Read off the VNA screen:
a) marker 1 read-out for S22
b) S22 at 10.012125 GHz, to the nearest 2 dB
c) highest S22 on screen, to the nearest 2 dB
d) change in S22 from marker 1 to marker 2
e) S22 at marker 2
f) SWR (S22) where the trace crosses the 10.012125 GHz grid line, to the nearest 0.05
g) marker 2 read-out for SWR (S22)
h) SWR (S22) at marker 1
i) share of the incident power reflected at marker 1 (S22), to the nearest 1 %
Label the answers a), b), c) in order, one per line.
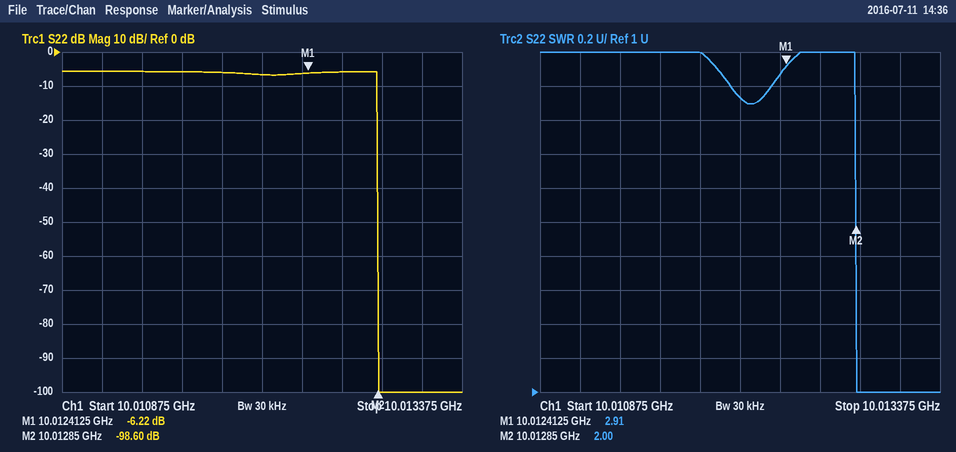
a) -6.22 dB
b) -6 dB
c) -6 dB
d) -92.38 dB
e) -98.60 dB
f) 2.75
g) 2.00
h) 2.91
i) 24 %
